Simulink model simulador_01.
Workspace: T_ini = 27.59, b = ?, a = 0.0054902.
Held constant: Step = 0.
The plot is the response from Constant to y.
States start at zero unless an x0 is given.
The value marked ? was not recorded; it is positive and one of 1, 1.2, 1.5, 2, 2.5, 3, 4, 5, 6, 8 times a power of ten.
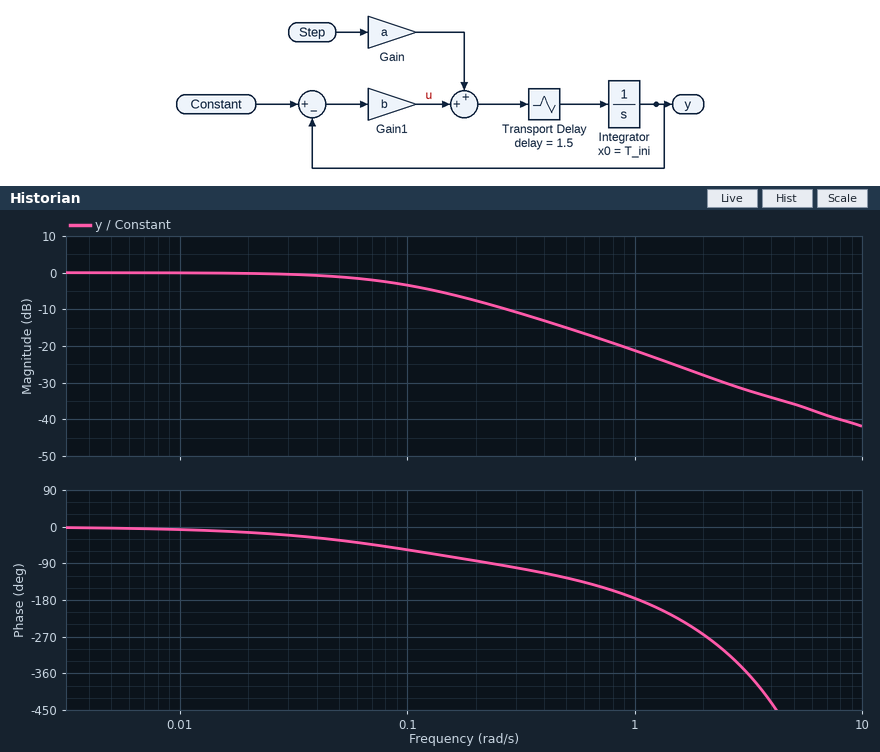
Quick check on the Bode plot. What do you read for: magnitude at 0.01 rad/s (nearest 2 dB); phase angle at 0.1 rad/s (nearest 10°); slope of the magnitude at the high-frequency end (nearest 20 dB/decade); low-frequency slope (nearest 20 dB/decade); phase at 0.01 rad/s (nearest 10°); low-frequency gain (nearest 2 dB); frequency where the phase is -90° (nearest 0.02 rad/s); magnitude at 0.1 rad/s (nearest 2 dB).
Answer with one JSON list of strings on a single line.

["0 dB", "-60°", "-20 dB/decade", "0 dB/decade", "-10°", "0 dB", "0.24 rad/s", "-4 dB"]
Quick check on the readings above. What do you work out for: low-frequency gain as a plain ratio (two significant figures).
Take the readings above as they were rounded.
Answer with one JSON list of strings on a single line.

["1.0"]
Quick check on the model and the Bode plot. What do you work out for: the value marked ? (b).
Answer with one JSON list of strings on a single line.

["0.08"]
